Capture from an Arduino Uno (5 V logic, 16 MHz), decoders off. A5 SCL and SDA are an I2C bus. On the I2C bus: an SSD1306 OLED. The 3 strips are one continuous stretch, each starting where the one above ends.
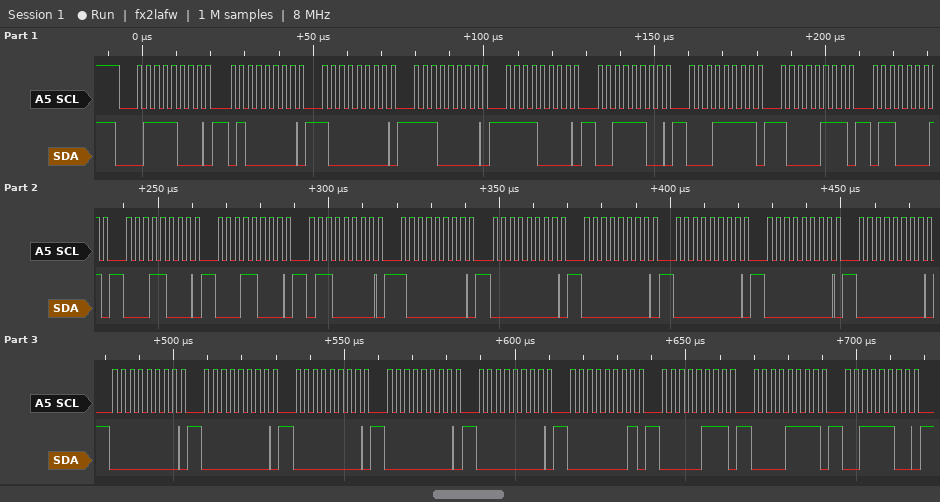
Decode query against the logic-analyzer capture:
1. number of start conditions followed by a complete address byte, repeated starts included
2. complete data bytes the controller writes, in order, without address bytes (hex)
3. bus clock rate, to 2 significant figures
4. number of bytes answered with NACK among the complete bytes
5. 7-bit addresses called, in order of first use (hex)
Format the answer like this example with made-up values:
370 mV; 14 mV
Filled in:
1; 40 80 E0 F0 3C 1F 87 61 18 18 60 80 00 00 00 00 00 00 00 00 00 00 01 07 0F 3C; 400 kHz; 0; 0x3C
